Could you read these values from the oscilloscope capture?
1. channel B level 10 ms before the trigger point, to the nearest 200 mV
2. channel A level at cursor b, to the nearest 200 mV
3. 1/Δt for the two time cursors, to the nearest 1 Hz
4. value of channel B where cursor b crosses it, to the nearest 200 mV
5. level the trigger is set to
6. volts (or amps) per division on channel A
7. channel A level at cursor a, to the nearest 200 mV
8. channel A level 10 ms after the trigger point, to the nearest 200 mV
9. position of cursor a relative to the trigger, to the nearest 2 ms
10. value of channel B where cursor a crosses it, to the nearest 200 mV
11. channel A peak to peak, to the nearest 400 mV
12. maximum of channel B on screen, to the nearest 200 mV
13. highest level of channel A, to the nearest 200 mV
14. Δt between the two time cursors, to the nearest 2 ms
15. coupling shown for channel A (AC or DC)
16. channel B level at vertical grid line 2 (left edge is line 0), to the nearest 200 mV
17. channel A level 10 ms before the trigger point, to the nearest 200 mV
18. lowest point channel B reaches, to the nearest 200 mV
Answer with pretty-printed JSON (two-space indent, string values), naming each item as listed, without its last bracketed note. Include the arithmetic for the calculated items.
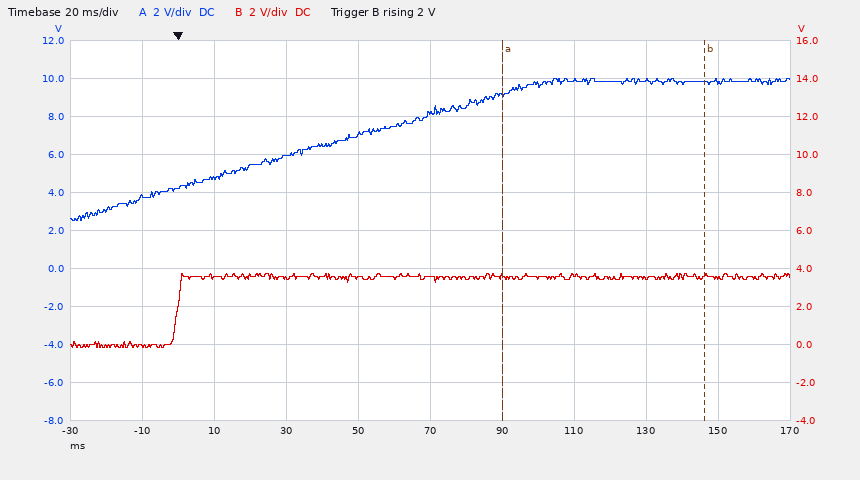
{
  "channel B level 10 ms before the trigger point, to the nearest 200 mV": "0.0 V",
  "channel A level at cursor b, to the nearest 200 mV": "9.8 V",
  "1/Δt for the two time cursors, to the nearest 1 Hz": "1 / 56 ms ≈ 18 Hz",
  "value of channel B where cursor b crosses it, to the nearest 200 mV": "3.6 V",
  "level the trigger is set to": "2 V",
  "volts (or amps) per division on channel A": "2 V",
  "channel A level at cursor a, to the nearest 200 mV": "9.2 V",
  "channel A level 10 ms after the trigger point, to the nearest 200 mV": "4.8 V",
  "position of cursor a relative to the trigger, to the nearest 2 ms": "+90 ms",
  "value of channel B where cursor a crosses it, to the nearest 200 mV": "3.6 V",
  "channel A peak to peak, to the nearest 400 mV": "7.6 V",
  "maximum of channel B on screen, to the nearest 200 mV": "3.8 V",
  "highest level of channel A, to the nearest 200 mV": "10.0 V",
  "Δt between the two time cursors, to the nearest 2 ms": "56 ms",
  "coupling shown for channel A": "DC",
  "channel B level at vertical grid line 2 (left edge is line 0), to the nearest 200 mV": "3.6 V",
  "channel A level 10 ms before the trigger point, to the nearest 200 mV": "3.8 V",
  "lowest point channel B reaches, to the nearest 200 mV": "-200 mV"
}
